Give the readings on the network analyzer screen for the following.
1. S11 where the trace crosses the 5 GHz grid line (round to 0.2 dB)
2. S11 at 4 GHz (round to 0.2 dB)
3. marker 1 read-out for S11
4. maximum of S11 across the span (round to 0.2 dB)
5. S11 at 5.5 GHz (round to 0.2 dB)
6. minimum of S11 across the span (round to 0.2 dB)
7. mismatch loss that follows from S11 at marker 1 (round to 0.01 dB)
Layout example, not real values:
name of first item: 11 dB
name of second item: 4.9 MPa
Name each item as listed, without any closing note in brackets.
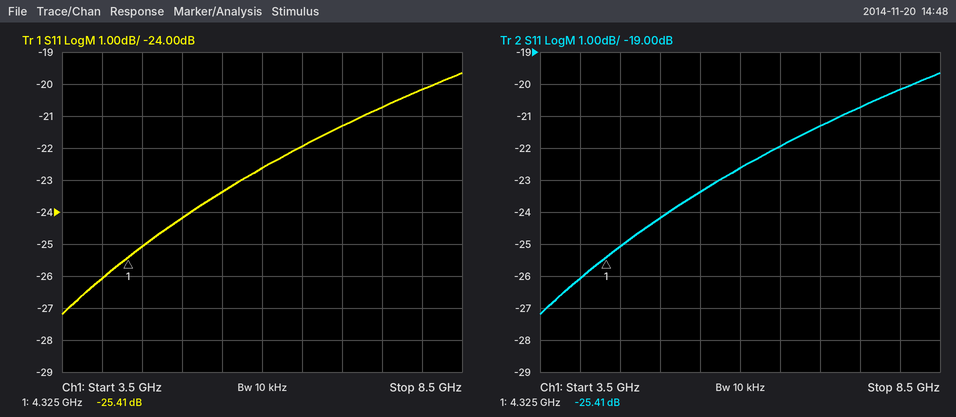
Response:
S11 where the trace crosses the 5 GHz grid line: -24.2 dB
S11 at 4 GHz: -26.0 dB
marker 1 read-out for S11: -25.41 dB
maximum of S11 across the span: -19.6 dB
S11 at 5.5 GHz: -23.4 dB
minimum of S11 across the span: -27.2 dB
mismatch loss that follows from S11 at marker 1: 0.01 dB
